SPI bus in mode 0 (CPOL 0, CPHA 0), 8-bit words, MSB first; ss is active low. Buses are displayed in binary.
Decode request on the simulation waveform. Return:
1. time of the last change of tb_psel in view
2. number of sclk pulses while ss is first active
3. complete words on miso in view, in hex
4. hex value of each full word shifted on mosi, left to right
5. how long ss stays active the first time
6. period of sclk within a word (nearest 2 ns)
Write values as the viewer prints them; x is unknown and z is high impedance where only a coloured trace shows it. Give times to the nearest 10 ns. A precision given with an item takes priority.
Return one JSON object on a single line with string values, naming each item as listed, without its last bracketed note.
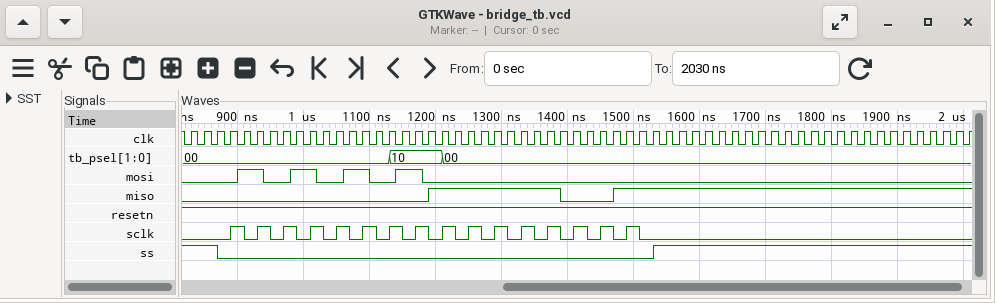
{"time of the last change of tb_psel in view": "1210 ns", "number of sclk pulses while ss is first active": "16", "complete words on miso in view, in hex": "00, F9", "hex value of each full word shifted on mosi, left to right": "55, 00", "how long ss stays active the first time": "660 ns", "period of sclk within a word": "40 ns"}
